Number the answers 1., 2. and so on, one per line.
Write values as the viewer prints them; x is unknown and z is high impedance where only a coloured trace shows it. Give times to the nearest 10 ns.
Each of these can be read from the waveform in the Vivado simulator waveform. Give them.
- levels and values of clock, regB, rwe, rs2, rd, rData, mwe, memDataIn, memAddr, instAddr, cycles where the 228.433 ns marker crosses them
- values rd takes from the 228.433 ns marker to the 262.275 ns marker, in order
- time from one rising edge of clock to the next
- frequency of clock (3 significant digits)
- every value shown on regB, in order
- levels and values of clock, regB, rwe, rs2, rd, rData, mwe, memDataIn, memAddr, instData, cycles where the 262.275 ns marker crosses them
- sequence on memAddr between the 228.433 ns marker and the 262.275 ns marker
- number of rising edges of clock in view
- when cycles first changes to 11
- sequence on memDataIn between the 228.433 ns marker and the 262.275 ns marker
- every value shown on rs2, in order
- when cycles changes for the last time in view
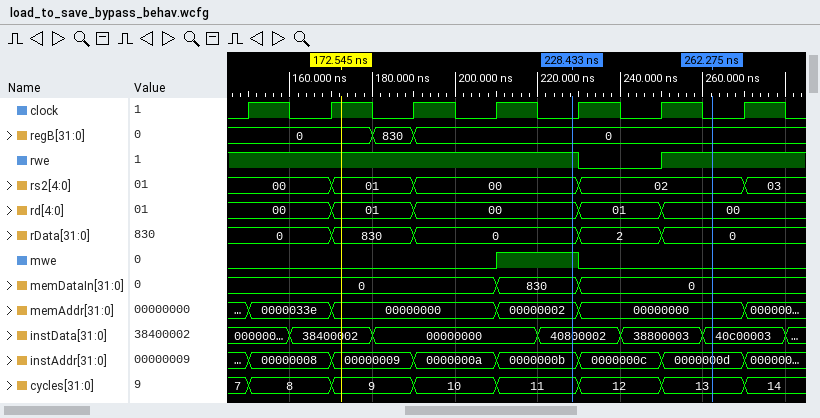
1. clock=0, regB=0, rwe=1, rs2=00, rd=00, rData=0, mwe=1, memDataIn=830, memAddr=00000002, instAddr=0000000b, cycles=11
2. 00, 01, 00
3. 20 ns
4. 50.0 MHz
5. 0, 830, 0
6. clock=0, regB=0, rwe=1, rs2=02, rd=00, rData=0, mwe=0, memDataIn=0, memAddr=00000000, instData=40c00003, cycles=13
7. 00000002, 00000000
8. 7
9. 210 ns
10. 830, 0
11. 00, 01, 00, 02, 03
12. 270 ns
